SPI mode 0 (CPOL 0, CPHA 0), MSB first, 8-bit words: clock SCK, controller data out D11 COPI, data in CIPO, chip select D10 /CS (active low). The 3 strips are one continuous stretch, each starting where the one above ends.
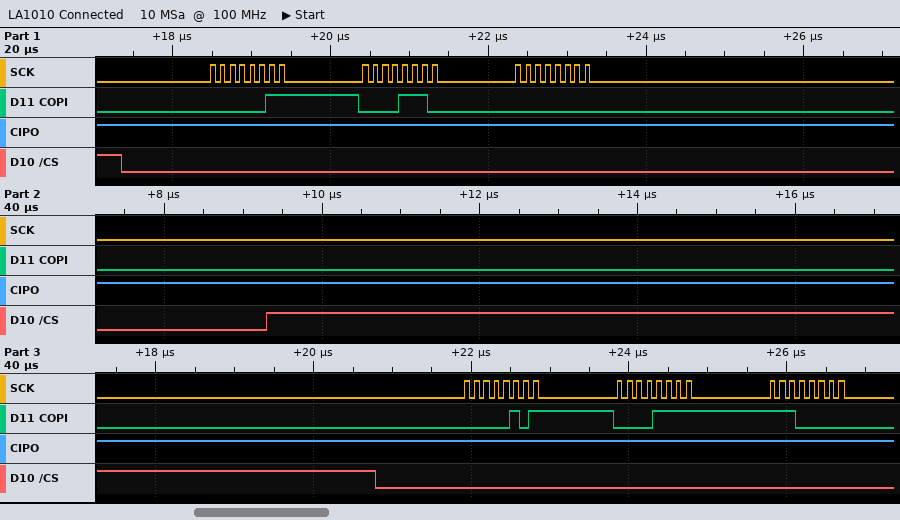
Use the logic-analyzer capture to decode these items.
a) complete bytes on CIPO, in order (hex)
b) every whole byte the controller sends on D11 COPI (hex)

0xFF 0xFF 0xFF 0xFF 0xFF 0xFF
0x03 0x0E 0x00 0x05 0x0F 0xE0
